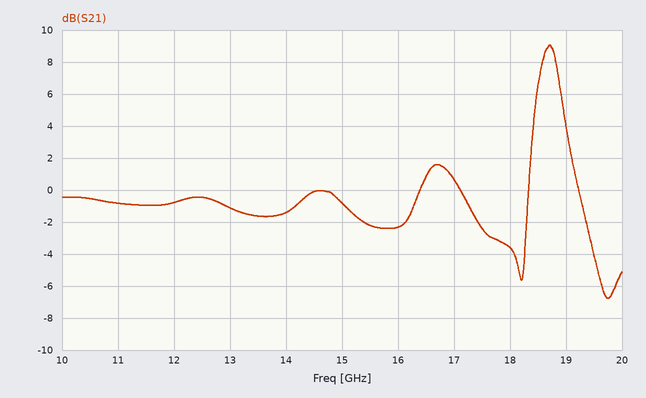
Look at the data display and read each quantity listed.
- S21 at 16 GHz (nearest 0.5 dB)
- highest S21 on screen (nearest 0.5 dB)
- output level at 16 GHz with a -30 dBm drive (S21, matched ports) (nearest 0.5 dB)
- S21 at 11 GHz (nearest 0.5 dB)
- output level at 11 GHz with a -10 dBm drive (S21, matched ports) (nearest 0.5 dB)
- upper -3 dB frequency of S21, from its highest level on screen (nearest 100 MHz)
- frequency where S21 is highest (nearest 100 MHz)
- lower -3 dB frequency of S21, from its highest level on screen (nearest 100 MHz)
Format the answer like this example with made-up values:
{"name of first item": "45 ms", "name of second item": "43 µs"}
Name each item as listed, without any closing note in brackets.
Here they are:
{"S21 at 16 GHz": "-2.5 dB", "highest S21 on screen": "9.0 dB", "output level at 16 GHz with a -30 dBm drive (S21, matched ports)": "-32.5 dBm", "S21 at 11 GHz": "-1.0 dB", "output level at 11 GHz with a -10 dBm drive (S21, matched ports)": "-11.0 dBm", "upper -3 dB frequency of S21, from its highest level on screen": "18.9 GHz", "frequency where S21 is highest": "18.7 GHz", "lower -3 dB frequency of S21, from its highest level on screen": "18.5 GHz"}
